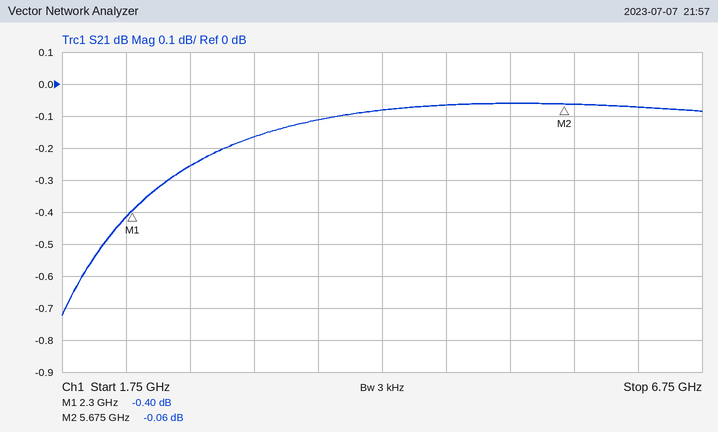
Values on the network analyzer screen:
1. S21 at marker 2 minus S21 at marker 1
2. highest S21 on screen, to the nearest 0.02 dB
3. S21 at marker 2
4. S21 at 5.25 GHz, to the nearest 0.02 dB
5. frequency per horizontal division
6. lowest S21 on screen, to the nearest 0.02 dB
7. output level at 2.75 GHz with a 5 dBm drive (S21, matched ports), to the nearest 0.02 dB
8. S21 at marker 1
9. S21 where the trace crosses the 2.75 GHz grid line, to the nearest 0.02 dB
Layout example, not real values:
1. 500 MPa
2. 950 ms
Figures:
1. 0.34 dB
2. -0.06 dB
3. -0.06 dB
4. -0.06 dB
5. 500 MHz
6. -0.72 dB
7. 4.74 dBm
8. -0.40 dB
9. -0.26 dB
